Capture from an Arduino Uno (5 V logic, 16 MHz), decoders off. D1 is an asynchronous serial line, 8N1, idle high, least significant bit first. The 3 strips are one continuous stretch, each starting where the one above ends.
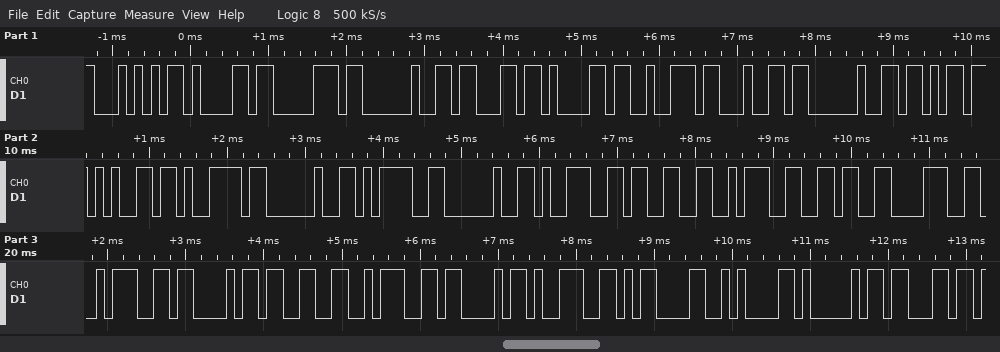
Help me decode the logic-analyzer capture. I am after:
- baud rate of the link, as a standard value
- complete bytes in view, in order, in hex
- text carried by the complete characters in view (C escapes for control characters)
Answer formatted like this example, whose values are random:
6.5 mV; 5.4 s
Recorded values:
9600 baud; 54 61 70 20 63 61 72 64 20 6B 65 79 20 3D 20 39 33 3A 36 38 3A 43 33 3A 43 39 0D 0A 41 63; "Tap card key = 93:68:C3:C9\r\nAc"
